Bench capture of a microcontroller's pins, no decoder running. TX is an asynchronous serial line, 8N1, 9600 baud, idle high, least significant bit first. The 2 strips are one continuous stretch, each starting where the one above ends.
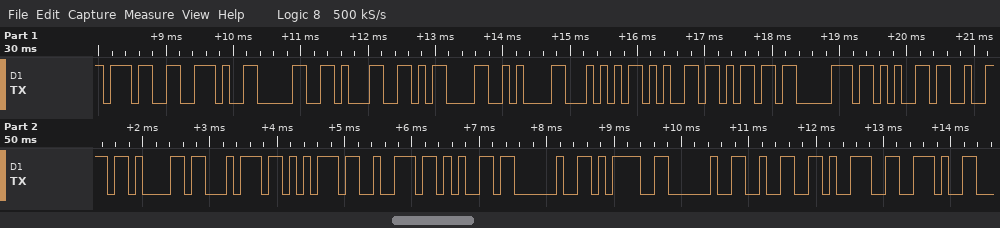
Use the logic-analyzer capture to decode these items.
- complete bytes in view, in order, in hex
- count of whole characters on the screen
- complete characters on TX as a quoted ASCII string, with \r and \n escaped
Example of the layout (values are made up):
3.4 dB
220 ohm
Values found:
37 2E 30 31 0D 0A 54 65 6D 70 65 72 61 74 75 72 65 20 3D 20 32 39 2E
23
"7.01\r\nTemperature = 29."
